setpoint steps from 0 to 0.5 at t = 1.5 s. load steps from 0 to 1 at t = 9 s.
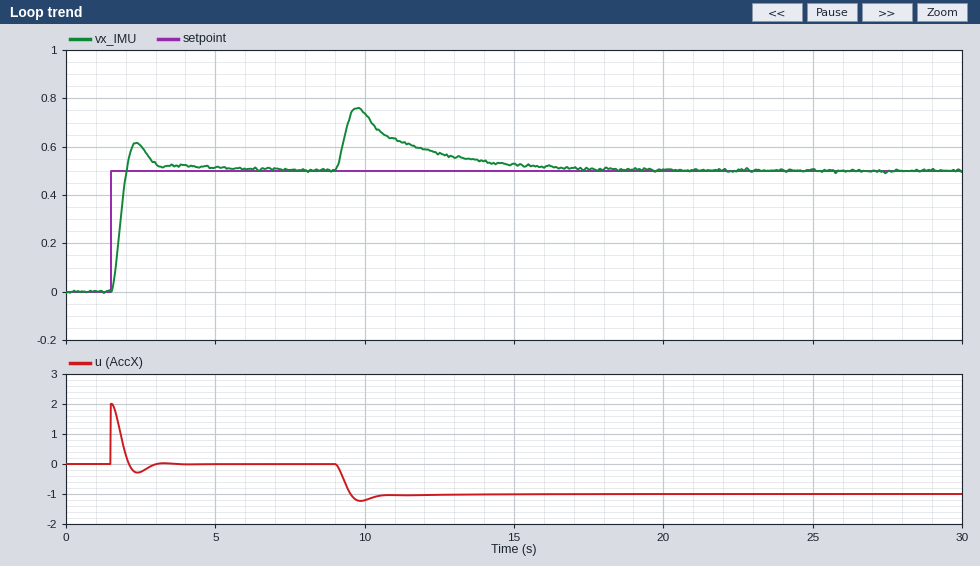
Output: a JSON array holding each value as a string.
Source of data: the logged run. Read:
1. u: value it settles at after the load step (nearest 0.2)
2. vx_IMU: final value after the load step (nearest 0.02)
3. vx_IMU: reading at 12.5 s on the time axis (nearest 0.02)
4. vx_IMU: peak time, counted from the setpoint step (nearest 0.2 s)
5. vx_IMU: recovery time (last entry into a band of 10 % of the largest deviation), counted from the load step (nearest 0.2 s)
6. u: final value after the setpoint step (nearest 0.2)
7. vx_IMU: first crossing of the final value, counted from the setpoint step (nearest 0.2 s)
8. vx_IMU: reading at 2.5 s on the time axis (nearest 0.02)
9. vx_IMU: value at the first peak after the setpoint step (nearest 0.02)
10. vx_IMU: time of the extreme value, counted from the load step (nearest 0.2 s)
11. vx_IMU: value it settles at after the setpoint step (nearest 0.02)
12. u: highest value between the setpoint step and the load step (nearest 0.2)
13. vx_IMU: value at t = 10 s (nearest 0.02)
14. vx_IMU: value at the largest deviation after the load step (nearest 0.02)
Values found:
["-1.0", "0.50", "0.58", "0.8 s", "6.0 s", "0.0", "0.6 s", "0.60", "0.62", "0.8 s", "0.50", "2.0", "0.74", "0.76"]
